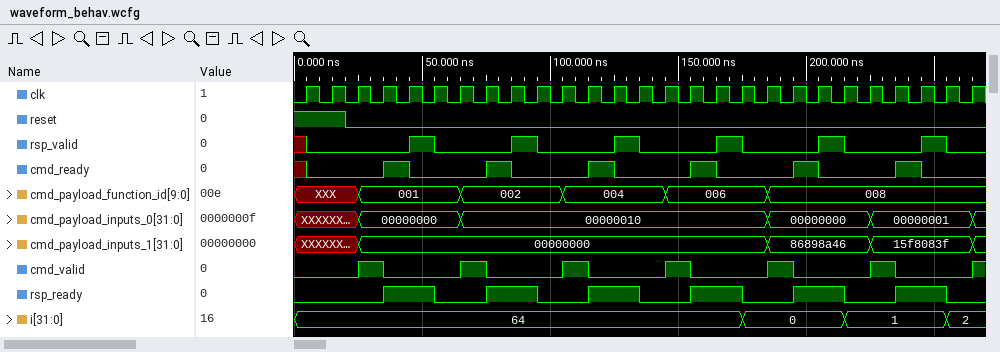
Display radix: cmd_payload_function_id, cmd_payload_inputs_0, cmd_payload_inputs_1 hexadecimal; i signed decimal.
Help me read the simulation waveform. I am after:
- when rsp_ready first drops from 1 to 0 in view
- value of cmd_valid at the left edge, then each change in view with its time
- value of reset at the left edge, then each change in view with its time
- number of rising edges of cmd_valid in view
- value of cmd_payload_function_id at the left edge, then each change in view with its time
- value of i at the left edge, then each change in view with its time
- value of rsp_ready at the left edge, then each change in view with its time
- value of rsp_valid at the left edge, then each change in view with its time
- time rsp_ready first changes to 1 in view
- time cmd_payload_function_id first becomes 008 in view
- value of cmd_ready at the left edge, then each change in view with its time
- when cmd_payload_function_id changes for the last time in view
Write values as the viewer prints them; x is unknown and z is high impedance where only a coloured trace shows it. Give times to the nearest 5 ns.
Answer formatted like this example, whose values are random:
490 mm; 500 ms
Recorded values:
55 ns; 0, 1 at 25 ns, 0 at 35 ns, 1 at 65 ns, 0 at 75 ns, 1 at 105 ns, 0 at 115 ns, 1 at 145 ns, 0 at 155 ns, 1 at 185 ns, 0 at 195 ns, 1 at 225 ns, 0 at 235 ns, 1 at 265 ns; 1, 0 at 20 ns; 7; XXX, 001 at 25 ns, 002 at 65 ns, 004 at 105 ns, 006 at 145 ns, 008 at 185 ns; 64, 0 at 175 ns, 1 at 215 ns, 2 at 255 ns; 0, 1 at 35 ns, 0 at 55 ns, 1 at 75 ns, 0 at 95 ns, 1 at 115 ns, 0 at 135 ns, 1 at 155 ns, 0 at 175 ns, 1 at 195 ns, 0 at 215 ns, 1 at 235 ns, 0 at 255 ns; x, 0 at 5 ns, 1 at 45 ns, 0 at 55 ns, 1 at 85 ns, 0 at 95 ns, 1 at 125 ns, 0 at 135 ns, 1 at 165 ns, 0 at 175 ns, 1 at 205 ns, 0 at 215 ns, 1 at 245 ns, 0 at 255 ns; 35 ns; 185 ns; x, 0 at 5 ns, 1 at 35 ns, 0 at 45 ns, 1 at 75 ns, 0 at 85 ns, 1 at 115 ns, 0 at 125 ns, 1 at 155 ns, 0 at 165 ns, 1 at 195 ns, 0 at 205 ns, 1 at 235 ns, 0 at 245 ns; 185 ns
